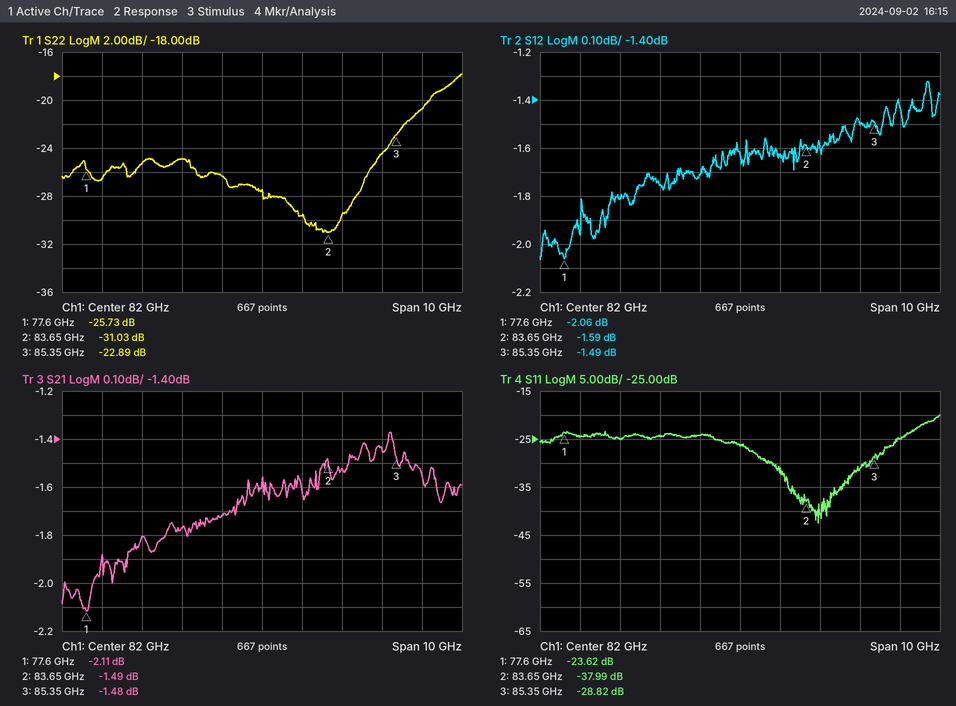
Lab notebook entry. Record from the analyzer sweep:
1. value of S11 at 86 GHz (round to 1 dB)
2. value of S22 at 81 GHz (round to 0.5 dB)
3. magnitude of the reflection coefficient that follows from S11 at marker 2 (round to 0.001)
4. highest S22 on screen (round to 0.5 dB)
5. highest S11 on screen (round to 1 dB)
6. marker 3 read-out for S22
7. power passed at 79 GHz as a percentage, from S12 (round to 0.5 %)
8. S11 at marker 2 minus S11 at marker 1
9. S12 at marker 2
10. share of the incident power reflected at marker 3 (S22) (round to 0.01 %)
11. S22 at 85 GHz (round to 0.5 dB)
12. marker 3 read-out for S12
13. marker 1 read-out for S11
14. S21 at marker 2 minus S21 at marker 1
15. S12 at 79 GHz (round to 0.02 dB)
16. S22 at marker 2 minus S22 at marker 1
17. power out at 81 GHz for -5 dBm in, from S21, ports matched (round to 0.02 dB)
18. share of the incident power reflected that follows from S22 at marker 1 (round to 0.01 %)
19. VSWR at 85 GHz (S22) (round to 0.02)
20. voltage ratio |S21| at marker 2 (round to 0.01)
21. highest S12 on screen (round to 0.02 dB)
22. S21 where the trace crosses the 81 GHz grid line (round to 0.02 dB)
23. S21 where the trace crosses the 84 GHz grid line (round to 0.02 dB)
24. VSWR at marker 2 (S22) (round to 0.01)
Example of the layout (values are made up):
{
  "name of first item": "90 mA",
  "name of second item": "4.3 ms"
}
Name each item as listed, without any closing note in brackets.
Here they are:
{
  "value of S11 at 86 GHz": "-25 dB",
  "value of S22 at 81 GHz": "-26.5 dB",
  "magnitude of the reflection coefficient that follows from S11 at marker 2": "0.013",
  "highest S22 on screen": "-18.0 dB",
  "highest S11 on screen": "-20 dB",
  "marker 3 read-out for S22": "-22.89 dB",
  "power passed at 79 GHz as a percentage, from S12": "66.0 %",
  "S11 at marker 2 minus S11 at marker 1": "-14.37 dB",
  "S12 at marker 2": "-1.59 dB",
  "share of the incident power reflected at marker 3 (S22)": "0.51 %",
  "S22 at 85 GHz": "-24.5 dB",
  "marker 3 read-out for S12": "-1.49 dB",
  "marker 1 read-out for S11": "-23.62 dB",
  "S21 at marker 2 minus S21 at marker 1": "0.62 dB",
  "S12 at 79 GHz": "-1.80 dB",
  "S22 at marker 2 minus S22 at marker 1": "-5.30 dB",
  "power out at 81 GHz for -5 dBm in, from S21, ports matched": "-6.72 dBm",
  "share of the incident power reflected that follows from S22 at marker 1": "0.27 %",
  "VSWR at 85 GHz (S22)": "1.12",
  "voltage ratio |S21| at marker 2": "0.84",
  "highest S12 on screen": "-1.32 dB",
  "S21 where the trace crosses the 81 GHz grid line": "-1.72 dB",
  "S21 where the trace crosses the 84 GHz grid line": "-1.52 dB",
  "VSWR at marker 2 (S22)": "1.06"
}
